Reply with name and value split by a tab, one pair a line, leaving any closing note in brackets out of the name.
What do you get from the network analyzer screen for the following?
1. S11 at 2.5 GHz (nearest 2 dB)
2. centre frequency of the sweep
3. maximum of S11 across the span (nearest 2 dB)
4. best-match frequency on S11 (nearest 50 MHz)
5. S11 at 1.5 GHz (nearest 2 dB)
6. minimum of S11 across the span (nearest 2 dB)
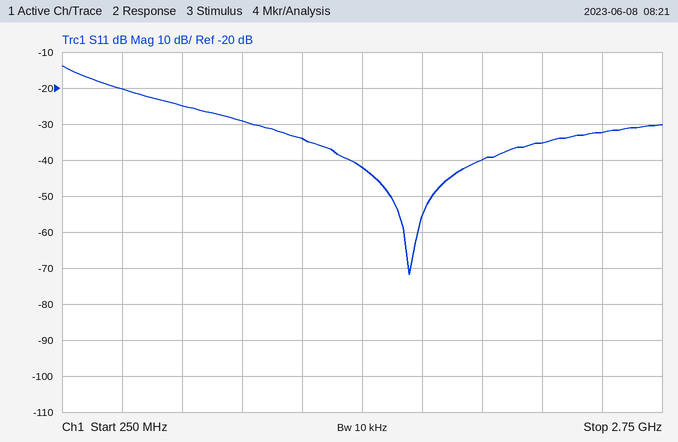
S11 at 2.5 GHz	-32 dB
centre frequency of the sweep	1.5 GHz
maximum of S11 across the span	-14 dB
best-match frequency on S11	1.70 GHz
S11 at 1.5 GHz	-42 dB
minimum of S11 across the span	-72 dB
